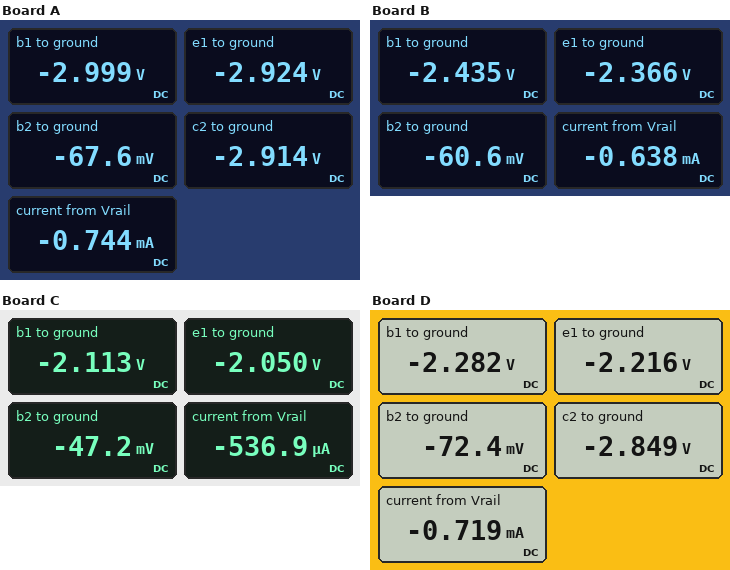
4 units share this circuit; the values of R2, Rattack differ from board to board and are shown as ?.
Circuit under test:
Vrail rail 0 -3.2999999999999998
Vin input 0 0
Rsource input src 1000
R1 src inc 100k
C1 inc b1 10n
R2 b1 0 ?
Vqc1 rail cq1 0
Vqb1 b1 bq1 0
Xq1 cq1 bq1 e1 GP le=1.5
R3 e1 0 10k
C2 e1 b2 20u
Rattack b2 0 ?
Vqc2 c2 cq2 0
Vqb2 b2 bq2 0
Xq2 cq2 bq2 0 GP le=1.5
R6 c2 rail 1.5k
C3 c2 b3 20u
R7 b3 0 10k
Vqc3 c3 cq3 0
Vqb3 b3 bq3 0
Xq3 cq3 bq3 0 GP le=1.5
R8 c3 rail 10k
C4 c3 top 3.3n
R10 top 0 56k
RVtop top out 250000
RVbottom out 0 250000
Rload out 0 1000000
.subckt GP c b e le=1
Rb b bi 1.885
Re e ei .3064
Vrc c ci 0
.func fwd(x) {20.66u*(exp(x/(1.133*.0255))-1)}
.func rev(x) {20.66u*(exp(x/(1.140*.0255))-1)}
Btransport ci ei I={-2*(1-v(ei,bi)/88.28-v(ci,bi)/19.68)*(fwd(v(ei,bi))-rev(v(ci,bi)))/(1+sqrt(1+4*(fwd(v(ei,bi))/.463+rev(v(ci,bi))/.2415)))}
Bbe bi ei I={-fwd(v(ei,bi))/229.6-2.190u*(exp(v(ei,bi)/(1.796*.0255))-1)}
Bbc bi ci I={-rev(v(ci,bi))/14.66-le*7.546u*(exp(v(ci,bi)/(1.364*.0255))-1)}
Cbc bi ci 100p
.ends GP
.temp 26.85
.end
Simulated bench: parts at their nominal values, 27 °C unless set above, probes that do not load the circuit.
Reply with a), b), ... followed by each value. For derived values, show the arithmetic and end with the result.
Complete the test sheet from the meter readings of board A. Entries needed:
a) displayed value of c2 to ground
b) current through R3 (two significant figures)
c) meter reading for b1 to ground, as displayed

a) -2.914 V
b) (0 V - (-2.924 V)) / 10 kΩ = 290 µA
c) -2.999 V
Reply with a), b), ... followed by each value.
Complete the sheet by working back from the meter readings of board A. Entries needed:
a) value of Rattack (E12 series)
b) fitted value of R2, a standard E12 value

a) 15 kΩ
b) 1.2 MΩ
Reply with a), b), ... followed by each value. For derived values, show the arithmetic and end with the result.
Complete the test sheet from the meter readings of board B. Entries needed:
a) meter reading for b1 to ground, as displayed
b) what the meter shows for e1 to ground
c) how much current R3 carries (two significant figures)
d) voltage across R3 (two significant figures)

a) -2.435 V
b) -2.366 V
c) (0 V - (-2.366 V)) / 10 kΩ = 240 µA
d) 0 V - (-2.366 V) = 2.4 V
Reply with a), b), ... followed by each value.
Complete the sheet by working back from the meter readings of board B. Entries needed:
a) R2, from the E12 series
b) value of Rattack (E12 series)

a) 560 kΩ
b) 10 kΩ
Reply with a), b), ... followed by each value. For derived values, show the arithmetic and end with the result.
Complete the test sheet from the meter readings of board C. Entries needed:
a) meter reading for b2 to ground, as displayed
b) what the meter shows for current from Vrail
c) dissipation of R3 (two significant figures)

a) -47.2 mV
b) -536.9 µA
c) (0 V - (-2.05 V))^2 / 10 kΩ = 420 µW
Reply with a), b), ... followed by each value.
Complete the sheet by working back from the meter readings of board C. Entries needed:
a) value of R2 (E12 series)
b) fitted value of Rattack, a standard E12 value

a) 390 kΩ
b) 5.6 kΩ
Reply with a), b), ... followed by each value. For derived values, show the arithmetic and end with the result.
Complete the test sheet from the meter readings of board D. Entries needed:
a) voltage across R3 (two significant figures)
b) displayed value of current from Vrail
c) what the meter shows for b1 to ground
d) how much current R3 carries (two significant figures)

a) 0 V - (-2.216 V) = 2.2 V
b) -0.719 mA
c) -2.282 V
d) (0 V - (-2.216 V)) / 10 kΩ = 220 µA
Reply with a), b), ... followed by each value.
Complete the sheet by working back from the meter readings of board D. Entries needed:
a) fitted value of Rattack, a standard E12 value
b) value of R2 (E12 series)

a) 22 kΩ
b) 470 kΩ
